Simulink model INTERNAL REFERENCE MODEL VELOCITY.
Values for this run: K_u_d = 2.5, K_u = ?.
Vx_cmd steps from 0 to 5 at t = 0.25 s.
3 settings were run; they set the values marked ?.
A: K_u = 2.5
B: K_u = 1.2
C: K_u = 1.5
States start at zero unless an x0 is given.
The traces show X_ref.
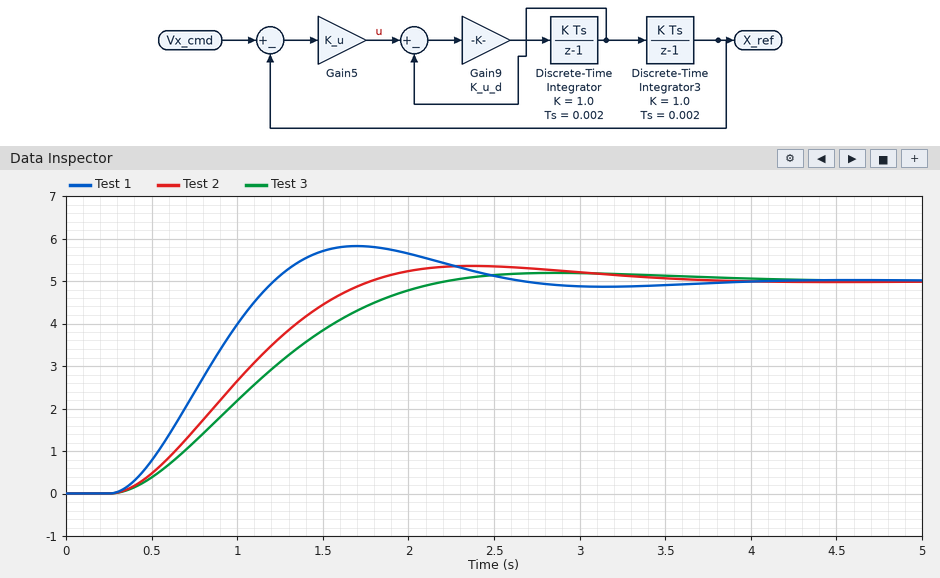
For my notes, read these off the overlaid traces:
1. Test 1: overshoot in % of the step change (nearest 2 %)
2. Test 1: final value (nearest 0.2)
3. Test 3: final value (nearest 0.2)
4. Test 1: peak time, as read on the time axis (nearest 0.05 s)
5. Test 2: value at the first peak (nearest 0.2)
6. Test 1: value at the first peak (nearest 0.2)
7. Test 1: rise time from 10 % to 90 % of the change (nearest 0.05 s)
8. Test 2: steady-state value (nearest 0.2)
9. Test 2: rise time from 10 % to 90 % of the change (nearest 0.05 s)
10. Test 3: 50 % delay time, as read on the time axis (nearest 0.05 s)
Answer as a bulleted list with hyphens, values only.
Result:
- 16 %
- 5.0
- 5.0
- 1.70 s
- 5.4
- 5.8
- 0.65 s
- 5.0
- 1.00 s
- 1.10 s
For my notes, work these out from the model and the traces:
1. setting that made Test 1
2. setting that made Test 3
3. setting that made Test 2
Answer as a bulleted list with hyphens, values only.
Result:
- A
- B
- C
